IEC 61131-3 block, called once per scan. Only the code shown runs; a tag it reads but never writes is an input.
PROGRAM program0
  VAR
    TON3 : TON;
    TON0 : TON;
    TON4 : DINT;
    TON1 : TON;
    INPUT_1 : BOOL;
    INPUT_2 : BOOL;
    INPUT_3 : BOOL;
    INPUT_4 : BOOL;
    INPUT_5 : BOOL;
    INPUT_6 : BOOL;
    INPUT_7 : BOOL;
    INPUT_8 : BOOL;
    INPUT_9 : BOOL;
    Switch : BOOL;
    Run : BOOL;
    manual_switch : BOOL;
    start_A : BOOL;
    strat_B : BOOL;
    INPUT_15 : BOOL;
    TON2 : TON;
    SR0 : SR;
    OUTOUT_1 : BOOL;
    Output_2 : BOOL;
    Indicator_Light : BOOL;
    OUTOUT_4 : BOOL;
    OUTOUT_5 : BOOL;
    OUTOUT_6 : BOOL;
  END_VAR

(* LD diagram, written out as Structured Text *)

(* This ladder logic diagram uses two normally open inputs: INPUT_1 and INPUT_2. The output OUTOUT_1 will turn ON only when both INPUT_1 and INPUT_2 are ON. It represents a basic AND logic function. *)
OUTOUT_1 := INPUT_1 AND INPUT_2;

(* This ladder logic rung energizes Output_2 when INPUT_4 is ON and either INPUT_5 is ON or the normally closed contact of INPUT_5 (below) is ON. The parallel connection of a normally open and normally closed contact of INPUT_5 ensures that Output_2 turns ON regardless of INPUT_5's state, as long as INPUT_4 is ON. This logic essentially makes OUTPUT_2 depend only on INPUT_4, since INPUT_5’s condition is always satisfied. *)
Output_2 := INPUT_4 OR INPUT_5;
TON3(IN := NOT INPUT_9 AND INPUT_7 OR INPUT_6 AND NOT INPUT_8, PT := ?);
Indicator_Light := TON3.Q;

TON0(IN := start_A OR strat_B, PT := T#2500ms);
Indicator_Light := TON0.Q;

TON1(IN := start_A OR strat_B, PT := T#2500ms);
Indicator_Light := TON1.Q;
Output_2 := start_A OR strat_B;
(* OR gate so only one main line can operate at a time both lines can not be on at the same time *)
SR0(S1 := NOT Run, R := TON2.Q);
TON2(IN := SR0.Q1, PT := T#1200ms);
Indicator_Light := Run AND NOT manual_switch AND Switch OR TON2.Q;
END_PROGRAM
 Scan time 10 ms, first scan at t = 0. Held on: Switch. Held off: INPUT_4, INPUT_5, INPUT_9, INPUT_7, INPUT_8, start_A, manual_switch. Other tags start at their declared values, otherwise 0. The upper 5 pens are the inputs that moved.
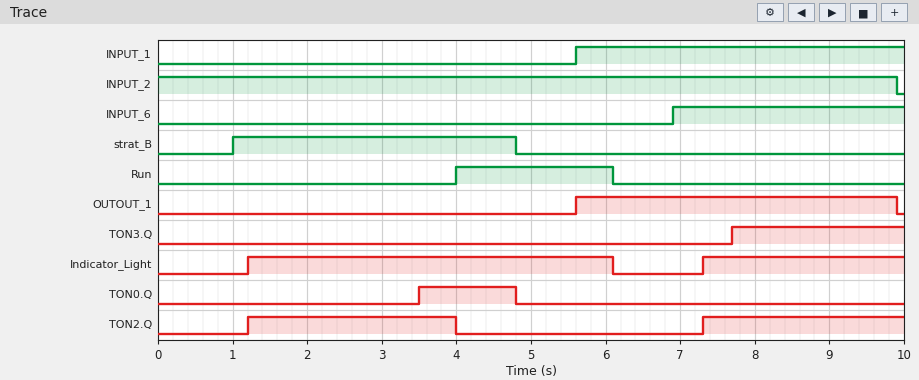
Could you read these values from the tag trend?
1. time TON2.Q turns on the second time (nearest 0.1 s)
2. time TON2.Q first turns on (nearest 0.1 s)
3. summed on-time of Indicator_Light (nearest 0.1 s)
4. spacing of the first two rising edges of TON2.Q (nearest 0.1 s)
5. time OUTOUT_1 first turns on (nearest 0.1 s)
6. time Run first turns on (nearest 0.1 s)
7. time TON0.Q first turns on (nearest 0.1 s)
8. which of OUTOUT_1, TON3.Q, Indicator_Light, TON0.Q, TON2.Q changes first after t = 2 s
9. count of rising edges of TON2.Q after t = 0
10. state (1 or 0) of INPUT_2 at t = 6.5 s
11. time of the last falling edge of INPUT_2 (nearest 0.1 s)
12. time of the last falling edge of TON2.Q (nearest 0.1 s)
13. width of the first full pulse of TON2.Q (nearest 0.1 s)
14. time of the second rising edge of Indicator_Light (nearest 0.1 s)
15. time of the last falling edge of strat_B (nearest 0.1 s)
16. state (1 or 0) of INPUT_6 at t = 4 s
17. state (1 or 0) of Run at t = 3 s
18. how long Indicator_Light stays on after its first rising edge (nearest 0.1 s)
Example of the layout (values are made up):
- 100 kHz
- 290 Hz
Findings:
- 7.3 s
- 1.2 s
- 7.6 s
- 6.1 s
- 5.6 s
- 4.0 s
- 3.5 s
- TON0.Q
- 2
- 1
- 9.9 s
- 4.0 s
- 2.8 s
- 7.3 s
- 4.8 s
- 0
- 0
- 4.9 s
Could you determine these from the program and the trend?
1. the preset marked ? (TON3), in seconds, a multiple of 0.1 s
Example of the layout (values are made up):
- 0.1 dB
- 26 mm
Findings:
- 0.8 s
